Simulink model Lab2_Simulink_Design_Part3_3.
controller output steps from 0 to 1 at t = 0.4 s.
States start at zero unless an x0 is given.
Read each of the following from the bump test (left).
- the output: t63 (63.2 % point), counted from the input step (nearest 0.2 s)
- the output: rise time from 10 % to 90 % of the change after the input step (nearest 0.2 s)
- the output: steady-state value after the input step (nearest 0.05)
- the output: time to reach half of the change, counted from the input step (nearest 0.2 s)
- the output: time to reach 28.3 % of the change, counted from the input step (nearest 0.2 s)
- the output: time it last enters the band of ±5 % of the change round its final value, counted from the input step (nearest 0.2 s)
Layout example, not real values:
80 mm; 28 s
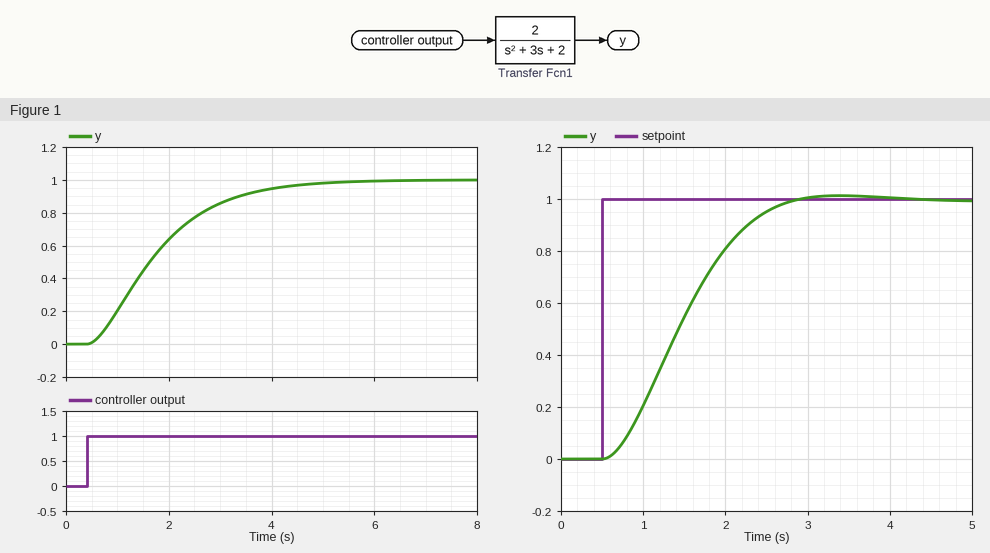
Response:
1.6 s; 2.6 s; 1.00; 1.2 s; 0.8 s; 3.6 s
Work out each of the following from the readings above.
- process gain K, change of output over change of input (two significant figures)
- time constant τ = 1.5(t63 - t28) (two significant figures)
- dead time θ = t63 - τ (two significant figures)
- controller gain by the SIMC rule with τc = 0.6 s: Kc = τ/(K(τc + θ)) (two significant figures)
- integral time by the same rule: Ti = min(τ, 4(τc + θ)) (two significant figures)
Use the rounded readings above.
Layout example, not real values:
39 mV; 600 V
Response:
1.0; 1.2 s; 0.40 s; 1.2; 1.2 s
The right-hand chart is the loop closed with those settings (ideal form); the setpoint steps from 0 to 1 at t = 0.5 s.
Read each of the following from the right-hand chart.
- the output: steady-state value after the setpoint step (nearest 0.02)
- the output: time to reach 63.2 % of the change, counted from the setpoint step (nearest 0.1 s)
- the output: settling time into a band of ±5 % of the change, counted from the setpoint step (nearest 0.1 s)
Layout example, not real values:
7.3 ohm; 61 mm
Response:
1.00; 1.1 s; 2.0 s
